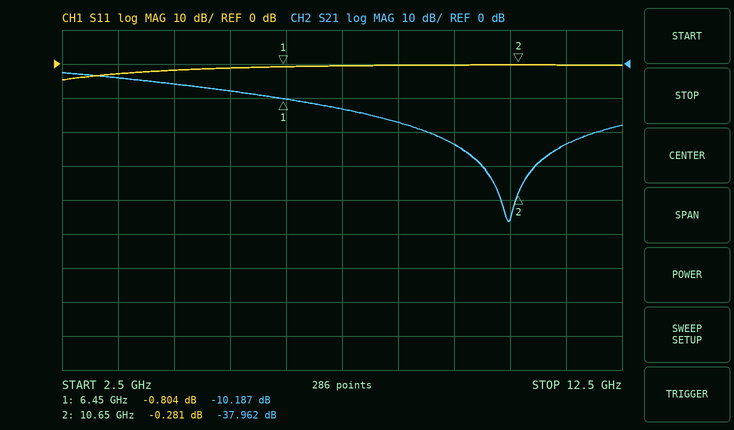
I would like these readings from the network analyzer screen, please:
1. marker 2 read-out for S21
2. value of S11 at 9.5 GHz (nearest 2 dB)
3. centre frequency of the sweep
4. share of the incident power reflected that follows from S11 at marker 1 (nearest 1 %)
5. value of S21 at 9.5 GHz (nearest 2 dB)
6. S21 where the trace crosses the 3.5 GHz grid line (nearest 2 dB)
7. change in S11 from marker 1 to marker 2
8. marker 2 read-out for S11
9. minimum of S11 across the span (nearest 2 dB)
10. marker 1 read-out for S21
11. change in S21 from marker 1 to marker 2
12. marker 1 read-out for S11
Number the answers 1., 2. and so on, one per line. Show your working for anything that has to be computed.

1. -37.962 dB
2. 0 dB
3. 7.5 GHz
4. 10^(-0.804/10) ≈ 83 %
5. -24 dB
6. -4 dB
7. -0.281 − (-0.804) = 0.523 dB
8. -0.281 dB
9. -4 dB
10. -10.187 dB
11. -37.962 − (-10.187) = -27.775 dB
12. -0.804 dB
